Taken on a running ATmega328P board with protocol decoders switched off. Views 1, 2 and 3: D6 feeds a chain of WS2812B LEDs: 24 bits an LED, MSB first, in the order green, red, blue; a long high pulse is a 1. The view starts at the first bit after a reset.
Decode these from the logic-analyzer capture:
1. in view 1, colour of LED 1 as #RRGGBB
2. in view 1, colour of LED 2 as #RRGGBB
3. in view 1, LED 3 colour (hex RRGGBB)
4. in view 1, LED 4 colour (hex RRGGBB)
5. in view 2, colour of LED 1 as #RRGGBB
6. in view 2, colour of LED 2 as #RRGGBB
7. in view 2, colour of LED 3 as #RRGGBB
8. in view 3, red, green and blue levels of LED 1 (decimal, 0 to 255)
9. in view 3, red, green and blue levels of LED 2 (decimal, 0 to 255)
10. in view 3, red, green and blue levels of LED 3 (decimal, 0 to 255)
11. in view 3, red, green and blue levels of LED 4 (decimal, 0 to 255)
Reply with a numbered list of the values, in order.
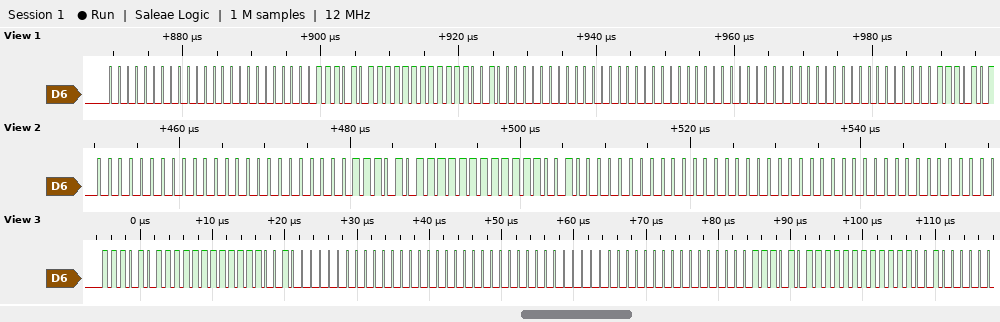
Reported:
1. #000000
2. #FFEBC8
3. #000000
4. #000000
5. #000000
6. #FFEBC8
7. #000000
8. 255, 235, 200
9. 0, 0, 0
10. 0, 0, 0
11. 255, 235, 200
